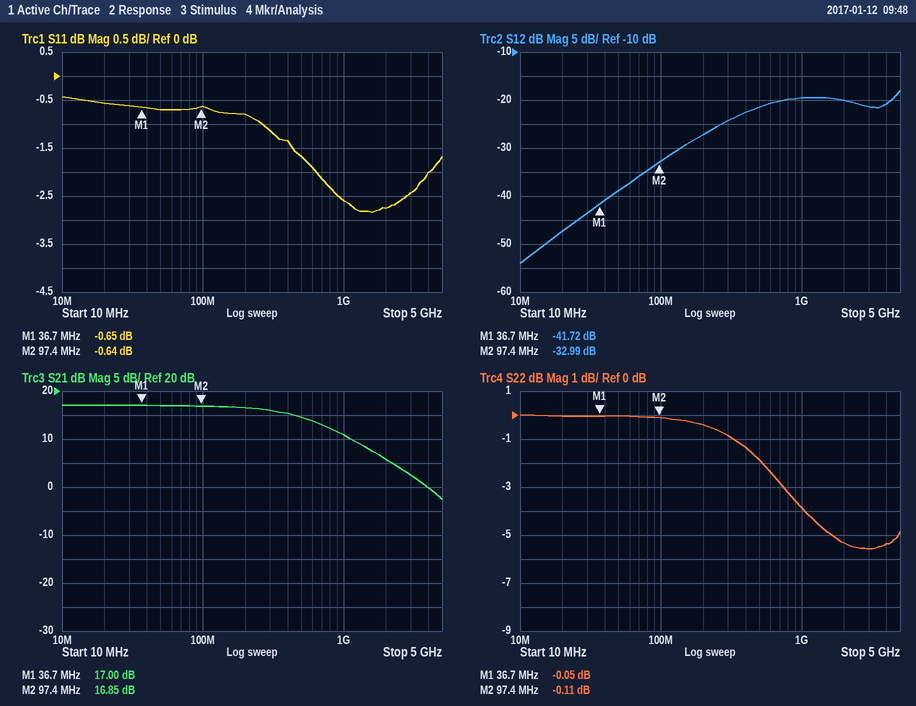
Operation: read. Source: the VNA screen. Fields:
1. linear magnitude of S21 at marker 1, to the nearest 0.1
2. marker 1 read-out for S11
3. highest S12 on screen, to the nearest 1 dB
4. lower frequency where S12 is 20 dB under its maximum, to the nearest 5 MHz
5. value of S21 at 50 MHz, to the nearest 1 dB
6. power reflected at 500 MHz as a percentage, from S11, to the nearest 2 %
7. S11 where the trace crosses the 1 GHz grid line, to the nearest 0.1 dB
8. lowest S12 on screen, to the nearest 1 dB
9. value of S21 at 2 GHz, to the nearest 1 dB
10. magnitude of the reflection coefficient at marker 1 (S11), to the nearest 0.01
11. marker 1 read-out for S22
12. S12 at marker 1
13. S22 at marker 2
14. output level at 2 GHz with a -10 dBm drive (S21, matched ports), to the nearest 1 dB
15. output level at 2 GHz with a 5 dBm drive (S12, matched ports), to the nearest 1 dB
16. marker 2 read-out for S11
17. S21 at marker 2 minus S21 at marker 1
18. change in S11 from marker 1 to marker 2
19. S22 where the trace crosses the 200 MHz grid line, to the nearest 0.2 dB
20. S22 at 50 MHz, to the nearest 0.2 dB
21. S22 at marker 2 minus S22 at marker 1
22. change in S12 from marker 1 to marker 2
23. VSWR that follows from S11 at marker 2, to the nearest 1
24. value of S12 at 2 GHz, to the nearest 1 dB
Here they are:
7.1
-0.65 dB
-18 dB
55 MHz
17 dB
68 %
-2.6 dB
-54 dB
6 dB
0.93
-0.05 dB
-41.72 dB
-0.11 dB
-4 dBm
-15 dBm
-0.64 dB
-0.15 dB
0.01 dB
-0.4 dB
0.0 dB
-0.06 dB
8.73 dB
27
-20 dB
